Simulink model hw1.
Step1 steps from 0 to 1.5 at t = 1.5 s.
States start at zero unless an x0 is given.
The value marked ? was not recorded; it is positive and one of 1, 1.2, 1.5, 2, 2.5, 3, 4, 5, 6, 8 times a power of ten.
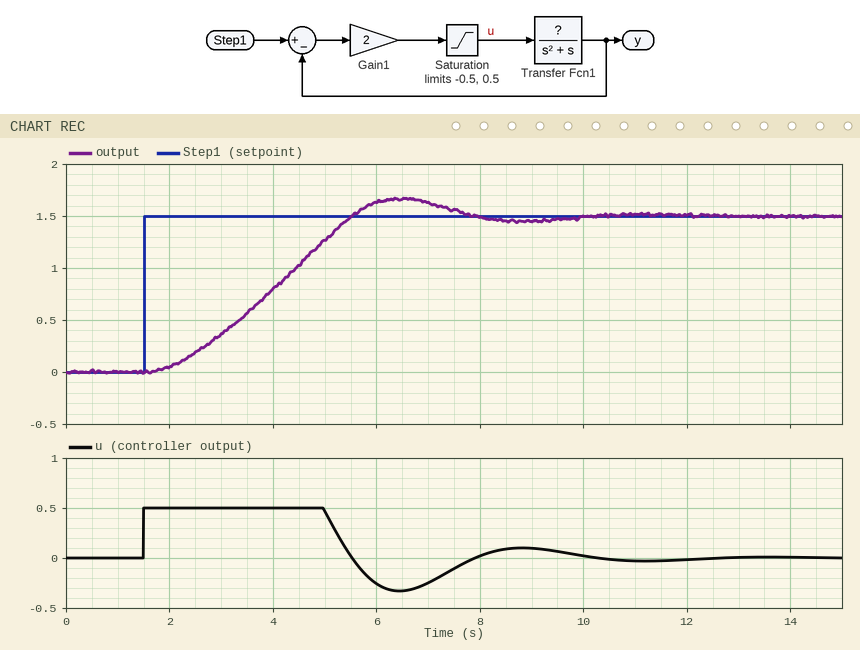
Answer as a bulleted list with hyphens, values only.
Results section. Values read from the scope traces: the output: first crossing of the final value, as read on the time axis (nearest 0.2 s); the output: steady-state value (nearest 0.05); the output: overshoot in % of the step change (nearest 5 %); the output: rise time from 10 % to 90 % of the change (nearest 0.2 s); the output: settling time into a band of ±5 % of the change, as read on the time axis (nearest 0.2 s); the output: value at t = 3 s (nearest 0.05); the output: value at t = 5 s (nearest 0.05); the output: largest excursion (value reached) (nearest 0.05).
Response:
- 5.6 s
- 1.50
- 10 %
- 2.8 s
- 7.4 s
- 0.35
- 1.25
- 1.65
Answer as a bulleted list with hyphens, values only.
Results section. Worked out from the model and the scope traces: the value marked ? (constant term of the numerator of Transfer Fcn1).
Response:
- 1
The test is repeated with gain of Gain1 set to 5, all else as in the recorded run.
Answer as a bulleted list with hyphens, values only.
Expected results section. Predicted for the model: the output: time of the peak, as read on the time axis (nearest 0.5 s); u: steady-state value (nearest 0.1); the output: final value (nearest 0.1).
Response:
- 6.0 s
- 0.0
- 1.5
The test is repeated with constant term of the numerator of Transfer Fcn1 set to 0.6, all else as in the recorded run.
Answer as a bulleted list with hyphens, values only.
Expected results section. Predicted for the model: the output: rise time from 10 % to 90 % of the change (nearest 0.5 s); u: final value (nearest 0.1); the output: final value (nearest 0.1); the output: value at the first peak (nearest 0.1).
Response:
- 4.5 s
- 0.0
- 1.5
- 1.6
